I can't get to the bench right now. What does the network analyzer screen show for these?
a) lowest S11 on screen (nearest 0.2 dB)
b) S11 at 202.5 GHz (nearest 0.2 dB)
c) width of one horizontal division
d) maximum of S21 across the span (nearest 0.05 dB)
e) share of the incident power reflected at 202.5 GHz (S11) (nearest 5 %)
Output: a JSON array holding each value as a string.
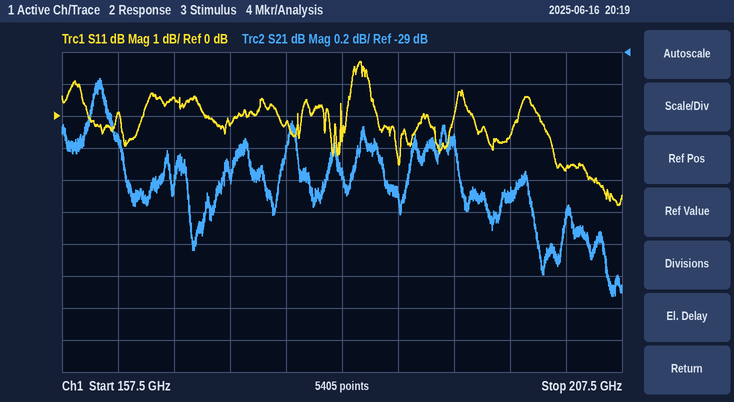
["-2.8 dB", "-1.6 dB", "5 GHz", "-29.15 dB", "70 %"]
